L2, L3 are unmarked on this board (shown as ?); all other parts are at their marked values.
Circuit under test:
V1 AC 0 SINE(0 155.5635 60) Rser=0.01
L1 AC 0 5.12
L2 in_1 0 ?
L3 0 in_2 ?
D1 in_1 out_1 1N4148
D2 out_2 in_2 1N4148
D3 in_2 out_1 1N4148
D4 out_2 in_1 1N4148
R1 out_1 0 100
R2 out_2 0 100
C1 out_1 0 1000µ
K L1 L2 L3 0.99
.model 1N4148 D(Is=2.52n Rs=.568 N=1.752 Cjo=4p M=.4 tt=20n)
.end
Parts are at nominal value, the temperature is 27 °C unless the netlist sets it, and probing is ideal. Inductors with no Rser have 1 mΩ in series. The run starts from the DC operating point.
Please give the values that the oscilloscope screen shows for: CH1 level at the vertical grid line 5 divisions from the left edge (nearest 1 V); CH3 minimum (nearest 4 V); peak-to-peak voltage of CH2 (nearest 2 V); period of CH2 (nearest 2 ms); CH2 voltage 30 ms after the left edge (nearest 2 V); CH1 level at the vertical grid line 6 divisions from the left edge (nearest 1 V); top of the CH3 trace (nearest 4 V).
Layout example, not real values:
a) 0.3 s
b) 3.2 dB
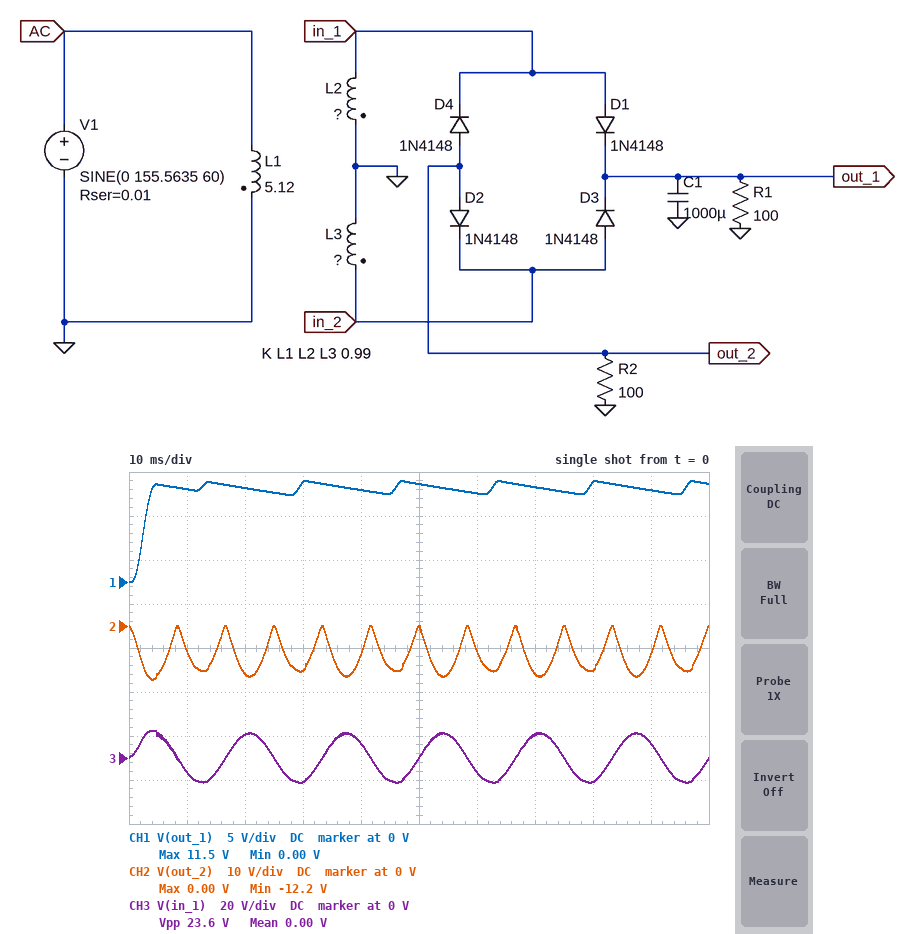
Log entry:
a) 11 V
b) -12 V
c) 12 V
d) 8 ms
e) -10 V
f) 10 V
g) 12 V
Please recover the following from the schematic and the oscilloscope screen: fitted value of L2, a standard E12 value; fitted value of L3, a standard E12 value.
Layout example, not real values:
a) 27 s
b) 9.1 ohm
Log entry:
a) 27 mH
b) 33 mH
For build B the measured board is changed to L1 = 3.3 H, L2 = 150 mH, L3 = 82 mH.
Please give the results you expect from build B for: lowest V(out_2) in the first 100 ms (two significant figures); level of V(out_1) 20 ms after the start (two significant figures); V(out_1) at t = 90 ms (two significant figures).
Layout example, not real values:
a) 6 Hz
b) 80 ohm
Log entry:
a) -32 V
b) 39 V
c) 30 V
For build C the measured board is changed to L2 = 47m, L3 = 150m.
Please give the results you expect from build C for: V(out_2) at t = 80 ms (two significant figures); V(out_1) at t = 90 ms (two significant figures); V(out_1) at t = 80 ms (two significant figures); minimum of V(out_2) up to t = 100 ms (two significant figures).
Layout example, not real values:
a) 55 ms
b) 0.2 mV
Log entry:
a) -13 V
b) 22 V
c) 23 V
d) -28 V
